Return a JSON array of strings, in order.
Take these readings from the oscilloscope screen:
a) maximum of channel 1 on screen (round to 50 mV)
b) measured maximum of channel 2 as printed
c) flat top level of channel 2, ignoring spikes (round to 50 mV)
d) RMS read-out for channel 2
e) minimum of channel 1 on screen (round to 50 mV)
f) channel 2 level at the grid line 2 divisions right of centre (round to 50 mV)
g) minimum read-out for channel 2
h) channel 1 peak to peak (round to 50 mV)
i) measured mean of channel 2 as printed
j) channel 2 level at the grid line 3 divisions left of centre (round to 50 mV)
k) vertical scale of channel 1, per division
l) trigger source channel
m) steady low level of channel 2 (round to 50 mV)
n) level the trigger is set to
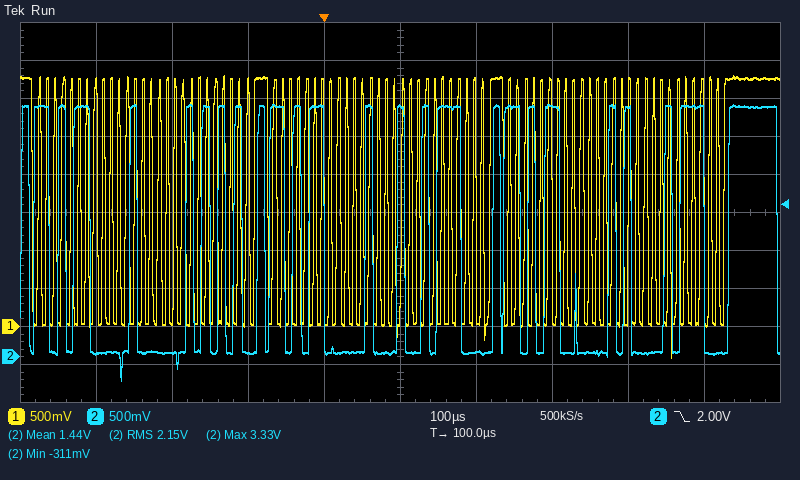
["3.30 V", "3.33 V", "3.30 V", "2.15 V", "-400 mV", "3.30 V", "-311 mV", "3.70 V", "1.44 V", "50 mV", "500 mV", "channel 2", "50 mV", "2.00 V"]
